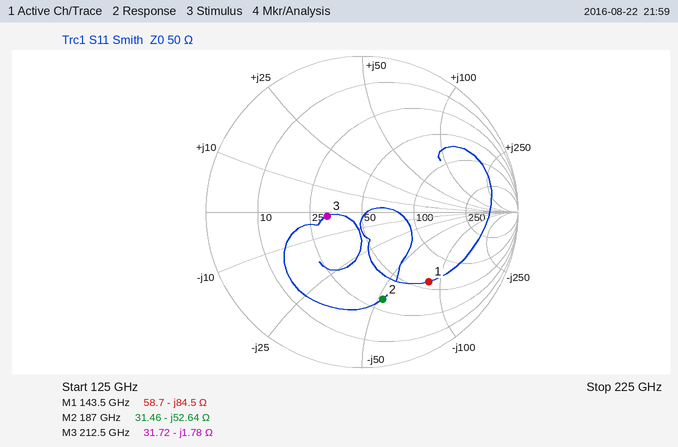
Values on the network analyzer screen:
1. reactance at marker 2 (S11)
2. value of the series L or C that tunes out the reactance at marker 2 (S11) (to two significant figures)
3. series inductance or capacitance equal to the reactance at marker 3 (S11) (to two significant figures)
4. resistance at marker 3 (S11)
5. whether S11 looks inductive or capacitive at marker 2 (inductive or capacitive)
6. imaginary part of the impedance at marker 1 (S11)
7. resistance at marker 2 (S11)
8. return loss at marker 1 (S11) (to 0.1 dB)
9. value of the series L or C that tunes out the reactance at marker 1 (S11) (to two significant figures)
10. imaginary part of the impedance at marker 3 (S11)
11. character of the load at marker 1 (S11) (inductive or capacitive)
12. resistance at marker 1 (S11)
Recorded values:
-52.64 Ω
45 pH
420 fF
31.72 Ω
capacitive
-84.5 Ω
31.46 Ω
4.2 dB
94 pH
-1.78 Ω
capacitive
58.7 Ω
